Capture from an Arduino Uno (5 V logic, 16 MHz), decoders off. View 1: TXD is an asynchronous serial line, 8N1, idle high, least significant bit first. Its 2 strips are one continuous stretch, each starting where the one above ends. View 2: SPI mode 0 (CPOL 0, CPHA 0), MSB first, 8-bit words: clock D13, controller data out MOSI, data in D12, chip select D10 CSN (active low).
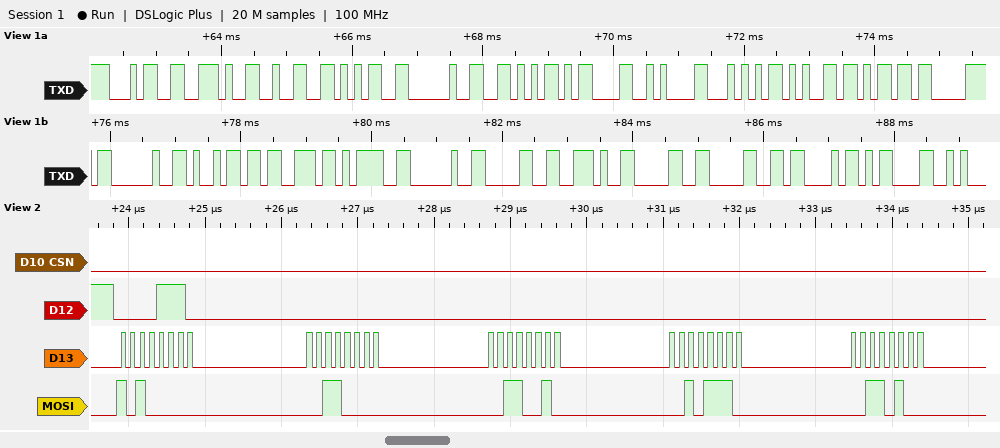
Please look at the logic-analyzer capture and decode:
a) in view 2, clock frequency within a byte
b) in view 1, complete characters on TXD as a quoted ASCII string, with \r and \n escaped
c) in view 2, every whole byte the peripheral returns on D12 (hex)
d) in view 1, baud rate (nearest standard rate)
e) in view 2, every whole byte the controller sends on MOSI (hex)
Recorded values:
8 MHz
"4.25 V\r\nTemp is= 0.00C\r"
0E 00 00 00 00
9600 baud
A0 30 32 2E 34
